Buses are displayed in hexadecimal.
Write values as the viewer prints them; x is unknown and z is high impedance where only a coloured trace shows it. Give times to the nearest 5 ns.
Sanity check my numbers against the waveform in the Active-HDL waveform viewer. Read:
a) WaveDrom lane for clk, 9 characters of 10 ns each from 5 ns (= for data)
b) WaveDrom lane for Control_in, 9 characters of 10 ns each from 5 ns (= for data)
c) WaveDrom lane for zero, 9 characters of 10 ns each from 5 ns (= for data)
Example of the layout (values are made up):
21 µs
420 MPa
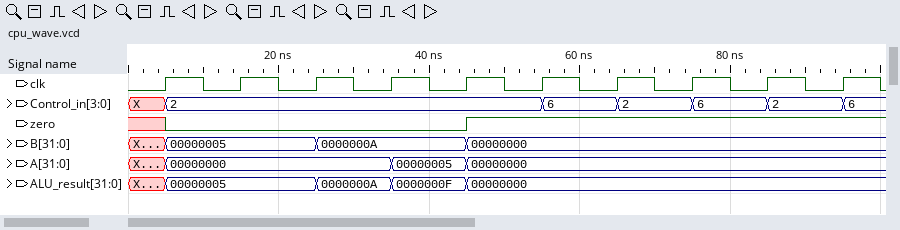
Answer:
{name: 'clk', wave: 'p........'}
{name: 'Control_in', wave: '=....====', data: '2 6 2 6 2'}
{name: 'zero', wave: '0...1....'}
